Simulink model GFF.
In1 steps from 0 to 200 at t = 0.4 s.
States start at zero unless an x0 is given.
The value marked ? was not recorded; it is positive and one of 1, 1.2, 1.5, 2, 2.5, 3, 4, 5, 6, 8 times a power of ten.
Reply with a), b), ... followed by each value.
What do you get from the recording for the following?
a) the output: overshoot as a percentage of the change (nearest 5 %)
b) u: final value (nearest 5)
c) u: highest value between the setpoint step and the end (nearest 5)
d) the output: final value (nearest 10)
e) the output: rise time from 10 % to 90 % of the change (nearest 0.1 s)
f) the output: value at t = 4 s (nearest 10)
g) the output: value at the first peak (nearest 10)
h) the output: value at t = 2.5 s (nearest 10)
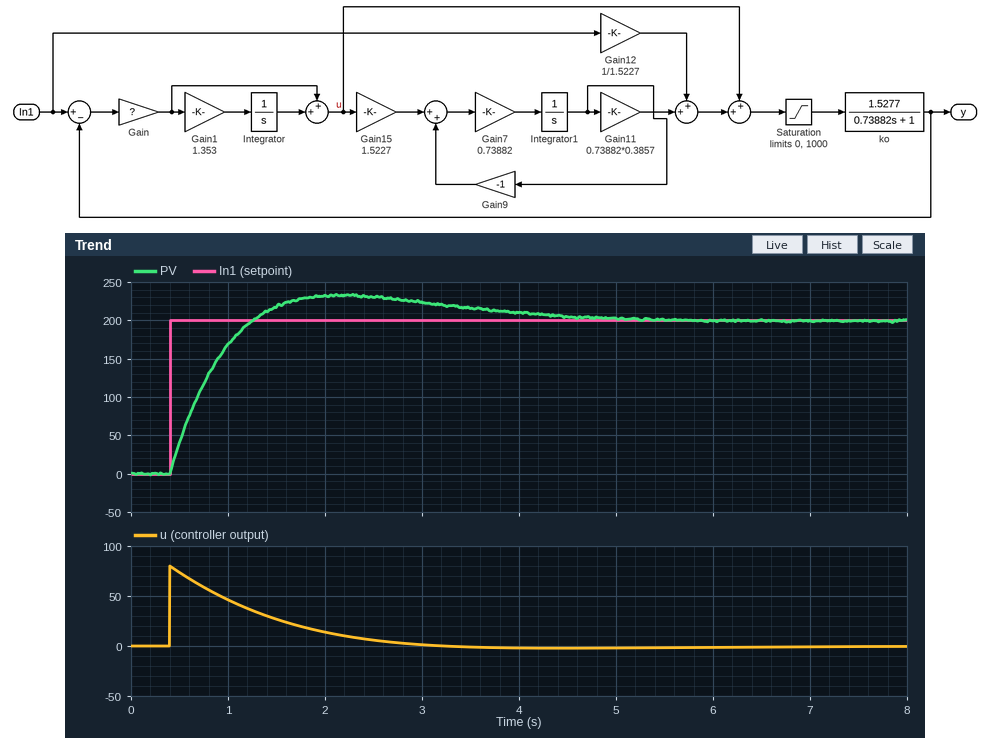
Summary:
a) 15 %
b) 0
c) 80
d) 200
e) 0.6 s
f) 210
g) 230
h) 230
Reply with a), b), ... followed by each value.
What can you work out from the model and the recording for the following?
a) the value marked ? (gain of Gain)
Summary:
a) 0.4
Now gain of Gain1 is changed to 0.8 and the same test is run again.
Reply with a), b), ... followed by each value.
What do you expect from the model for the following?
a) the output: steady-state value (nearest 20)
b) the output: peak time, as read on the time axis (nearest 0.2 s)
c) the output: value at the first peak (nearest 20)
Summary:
a) 200
b) 2.4 s
c) 220
